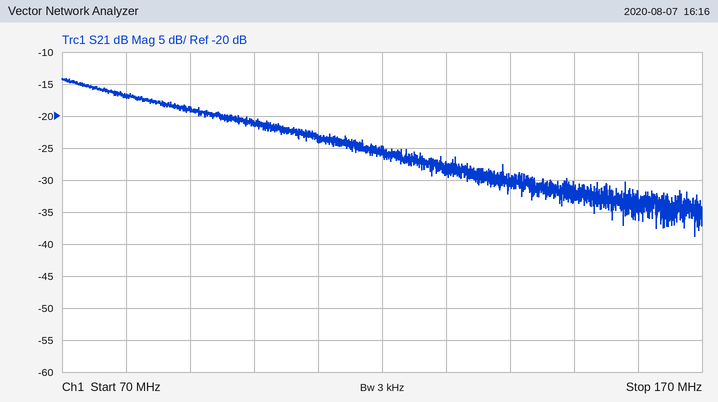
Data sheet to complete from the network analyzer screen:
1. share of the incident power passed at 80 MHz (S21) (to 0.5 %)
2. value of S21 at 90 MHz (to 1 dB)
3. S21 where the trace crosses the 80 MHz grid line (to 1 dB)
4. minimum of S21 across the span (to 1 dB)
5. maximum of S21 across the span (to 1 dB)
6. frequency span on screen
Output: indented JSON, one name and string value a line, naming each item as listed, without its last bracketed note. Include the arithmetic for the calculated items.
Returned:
{
  "share of the incident power passed at 80 MHz (S21)": "10^(-17/10) ≈ 2.0 %",
  "value of S21 at 90 MHz": "-19 dB",
  "S21 where the trace crosses the 80 MHz grid line": "-17 dB",
  "minimum of S21 across the span": "-39 dB",
  "maximum of S21 across the span": "-14 dB",
  "frequency span on screen": "100 MHz"
}
